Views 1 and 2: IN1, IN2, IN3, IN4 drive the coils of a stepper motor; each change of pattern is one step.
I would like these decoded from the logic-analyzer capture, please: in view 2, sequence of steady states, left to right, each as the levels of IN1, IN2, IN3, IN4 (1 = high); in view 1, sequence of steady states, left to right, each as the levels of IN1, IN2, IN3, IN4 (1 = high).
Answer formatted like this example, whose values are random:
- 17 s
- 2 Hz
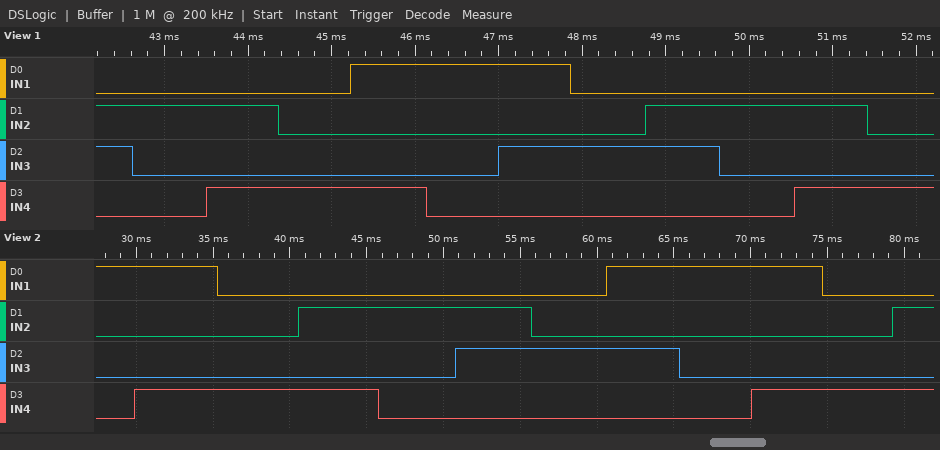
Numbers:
- 1000 1001 0001 0101 0100 0110 0010 1010 1000 1001 0001 0101
- 0110 0100 0101 0001 1001 1000 1010 0010 0110 0100 0101 0001
